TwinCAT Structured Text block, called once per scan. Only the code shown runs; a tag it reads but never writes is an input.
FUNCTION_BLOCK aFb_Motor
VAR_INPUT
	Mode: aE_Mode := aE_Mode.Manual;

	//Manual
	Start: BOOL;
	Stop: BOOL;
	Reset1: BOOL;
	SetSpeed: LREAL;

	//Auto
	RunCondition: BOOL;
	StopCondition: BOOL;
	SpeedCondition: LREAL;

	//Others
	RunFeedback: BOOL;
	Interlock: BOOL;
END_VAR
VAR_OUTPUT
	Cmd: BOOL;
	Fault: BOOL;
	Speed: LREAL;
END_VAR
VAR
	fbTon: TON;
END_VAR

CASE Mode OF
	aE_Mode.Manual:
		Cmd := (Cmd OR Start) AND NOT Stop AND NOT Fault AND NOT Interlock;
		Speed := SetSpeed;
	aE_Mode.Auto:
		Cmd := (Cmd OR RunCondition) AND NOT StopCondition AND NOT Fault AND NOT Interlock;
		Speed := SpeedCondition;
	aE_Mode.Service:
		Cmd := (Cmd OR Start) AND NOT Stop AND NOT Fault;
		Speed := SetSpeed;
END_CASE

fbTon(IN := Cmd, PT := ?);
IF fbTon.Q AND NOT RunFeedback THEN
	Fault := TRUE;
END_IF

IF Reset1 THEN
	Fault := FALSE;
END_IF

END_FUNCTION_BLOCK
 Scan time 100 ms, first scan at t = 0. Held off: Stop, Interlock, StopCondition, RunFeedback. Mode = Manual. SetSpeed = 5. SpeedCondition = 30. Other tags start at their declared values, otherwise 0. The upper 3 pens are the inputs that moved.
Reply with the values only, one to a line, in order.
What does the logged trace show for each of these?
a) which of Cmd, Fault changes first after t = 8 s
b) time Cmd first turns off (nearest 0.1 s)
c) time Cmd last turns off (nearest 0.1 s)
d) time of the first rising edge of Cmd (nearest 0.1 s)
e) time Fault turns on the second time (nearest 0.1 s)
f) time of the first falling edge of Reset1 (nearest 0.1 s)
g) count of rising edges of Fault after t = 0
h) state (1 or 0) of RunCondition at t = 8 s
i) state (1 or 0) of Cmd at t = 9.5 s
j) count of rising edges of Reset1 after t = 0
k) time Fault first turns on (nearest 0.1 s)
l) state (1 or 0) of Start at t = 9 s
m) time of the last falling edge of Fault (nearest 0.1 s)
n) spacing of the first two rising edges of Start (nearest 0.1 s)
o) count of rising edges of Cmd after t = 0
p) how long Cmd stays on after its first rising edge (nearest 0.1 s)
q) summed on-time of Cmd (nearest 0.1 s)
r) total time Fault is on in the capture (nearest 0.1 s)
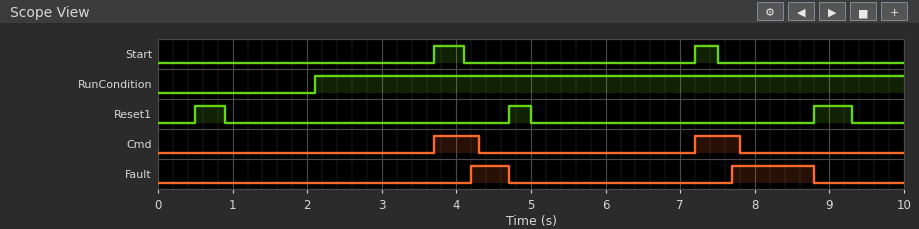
Fault
4.3 s
7.8 s
3.7 s
7.7 s
0.9 s
2
1
0
3
4.2 s
0
8.8 s
3.5 s
2
0.6 s
1.2 s
1.6 s
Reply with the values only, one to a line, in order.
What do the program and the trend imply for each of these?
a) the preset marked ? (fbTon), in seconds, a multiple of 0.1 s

0.5 s
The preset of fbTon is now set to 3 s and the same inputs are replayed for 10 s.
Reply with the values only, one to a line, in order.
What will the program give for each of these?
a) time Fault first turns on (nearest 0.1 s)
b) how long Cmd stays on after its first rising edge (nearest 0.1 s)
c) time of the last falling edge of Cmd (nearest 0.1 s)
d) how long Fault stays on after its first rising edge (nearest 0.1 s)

6.7 s
3.1 s
6.8 s
2.1 s
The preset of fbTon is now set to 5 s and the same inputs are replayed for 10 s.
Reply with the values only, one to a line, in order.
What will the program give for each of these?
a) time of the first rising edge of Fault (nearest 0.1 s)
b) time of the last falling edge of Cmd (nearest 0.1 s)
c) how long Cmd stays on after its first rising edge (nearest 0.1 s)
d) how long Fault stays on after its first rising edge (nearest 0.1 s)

8.7 s
8.8 s
5.1 s
0.1 s
